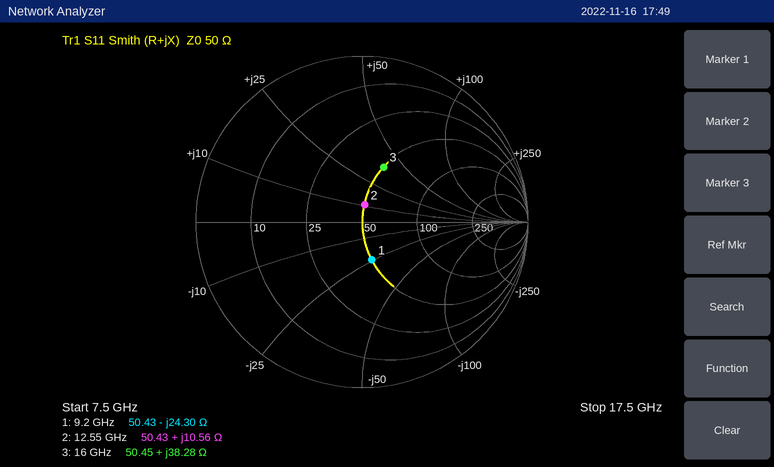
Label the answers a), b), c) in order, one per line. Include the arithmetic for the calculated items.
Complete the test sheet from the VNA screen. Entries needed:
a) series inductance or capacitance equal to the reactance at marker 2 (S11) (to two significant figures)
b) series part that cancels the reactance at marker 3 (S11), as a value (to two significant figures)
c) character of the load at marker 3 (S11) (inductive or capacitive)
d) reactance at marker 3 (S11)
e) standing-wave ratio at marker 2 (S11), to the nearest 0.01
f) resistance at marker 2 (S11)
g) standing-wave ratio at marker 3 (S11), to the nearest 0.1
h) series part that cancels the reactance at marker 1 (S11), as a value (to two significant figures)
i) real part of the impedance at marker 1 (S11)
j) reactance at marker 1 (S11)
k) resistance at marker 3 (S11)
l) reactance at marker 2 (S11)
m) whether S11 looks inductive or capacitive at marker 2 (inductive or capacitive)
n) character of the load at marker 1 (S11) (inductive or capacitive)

a) L = 10.56 Ω/(2π × 12.55 GHz) ≈ 134 pH, so 130 pH to two significant figures
b) C = 1/(2π × 16 GHz × 38.28 Ω) ≈ 260 fF
c) inductive
d) +38.28 Ω
e) 1.23
f) 50.43 Ω
g) 2.1
h) L = 24.3 Ω/(2π × 9.2 GHz) ≈ 420 pH
i) 50.43 Ω
j) -24.30 Ω
k) 50.45 Ω
l) +10.56 Ω
m) inductive
n) capacitive
